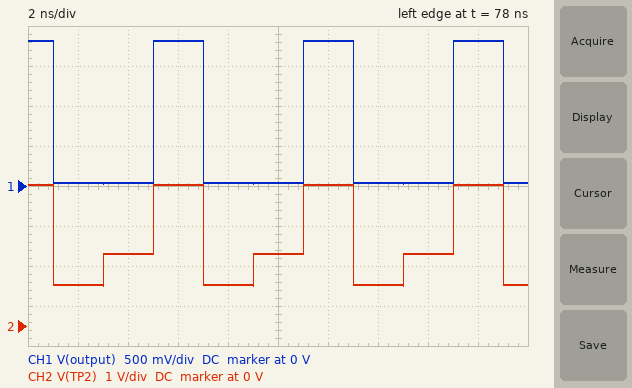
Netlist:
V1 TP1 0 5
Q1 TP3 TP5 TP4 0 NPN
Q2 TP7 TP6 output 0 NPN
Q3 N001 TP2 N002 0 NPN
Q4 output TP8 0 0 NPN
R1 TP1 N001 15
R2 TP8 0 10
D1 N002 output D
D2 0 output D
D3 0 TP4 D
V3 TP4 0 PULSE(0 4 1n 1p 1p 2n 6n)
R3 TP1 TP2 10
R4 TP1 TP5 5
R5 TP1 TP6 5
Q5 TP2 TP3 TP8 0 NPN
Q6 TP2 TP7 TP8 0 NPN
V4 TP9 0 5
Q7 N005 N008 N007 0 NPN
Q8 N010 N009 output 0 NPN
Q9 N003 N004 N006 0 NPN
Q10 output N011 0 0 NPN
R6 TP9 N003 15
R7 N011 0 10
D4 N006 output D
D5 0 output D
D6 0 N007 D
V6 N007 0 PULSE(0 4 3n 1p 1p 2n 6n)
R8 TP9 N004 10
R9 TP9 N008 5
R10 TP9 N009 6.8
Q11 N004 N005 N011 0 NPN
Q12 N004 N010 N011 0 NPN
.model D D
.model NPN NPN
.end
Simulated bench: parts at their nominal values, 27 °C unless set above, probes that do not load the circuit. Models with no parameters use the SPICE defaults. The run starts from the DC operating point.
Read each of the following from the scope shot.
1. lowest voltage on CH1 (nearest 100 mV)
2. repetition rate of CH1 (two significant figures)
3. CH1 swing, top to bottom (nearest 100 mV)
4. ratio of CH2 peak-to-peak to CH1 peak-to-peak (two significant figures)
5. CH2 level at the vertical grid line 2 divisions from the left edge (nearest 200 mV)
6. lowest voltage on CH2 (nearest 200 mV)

0 V
170 MHz
1.8 V
1.4
1.8 V
1.0 V
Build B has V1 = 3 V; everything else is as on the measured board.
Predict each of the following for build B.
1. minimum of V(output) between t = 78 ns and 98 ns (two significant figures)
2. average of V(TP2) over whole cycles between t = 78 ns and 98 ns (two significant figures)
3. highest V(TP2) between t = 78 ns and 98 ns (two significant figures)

26 mV
1.6 V
2.1 V
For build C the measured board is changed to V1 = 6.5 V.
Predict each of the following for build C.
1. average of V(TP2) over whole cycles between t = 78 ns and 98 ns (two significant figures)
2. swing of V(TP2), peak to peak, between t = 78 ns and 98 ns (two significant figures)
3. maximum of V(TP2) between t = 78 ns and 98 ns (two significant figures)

2.1 V
2.6 V
3.6 V
